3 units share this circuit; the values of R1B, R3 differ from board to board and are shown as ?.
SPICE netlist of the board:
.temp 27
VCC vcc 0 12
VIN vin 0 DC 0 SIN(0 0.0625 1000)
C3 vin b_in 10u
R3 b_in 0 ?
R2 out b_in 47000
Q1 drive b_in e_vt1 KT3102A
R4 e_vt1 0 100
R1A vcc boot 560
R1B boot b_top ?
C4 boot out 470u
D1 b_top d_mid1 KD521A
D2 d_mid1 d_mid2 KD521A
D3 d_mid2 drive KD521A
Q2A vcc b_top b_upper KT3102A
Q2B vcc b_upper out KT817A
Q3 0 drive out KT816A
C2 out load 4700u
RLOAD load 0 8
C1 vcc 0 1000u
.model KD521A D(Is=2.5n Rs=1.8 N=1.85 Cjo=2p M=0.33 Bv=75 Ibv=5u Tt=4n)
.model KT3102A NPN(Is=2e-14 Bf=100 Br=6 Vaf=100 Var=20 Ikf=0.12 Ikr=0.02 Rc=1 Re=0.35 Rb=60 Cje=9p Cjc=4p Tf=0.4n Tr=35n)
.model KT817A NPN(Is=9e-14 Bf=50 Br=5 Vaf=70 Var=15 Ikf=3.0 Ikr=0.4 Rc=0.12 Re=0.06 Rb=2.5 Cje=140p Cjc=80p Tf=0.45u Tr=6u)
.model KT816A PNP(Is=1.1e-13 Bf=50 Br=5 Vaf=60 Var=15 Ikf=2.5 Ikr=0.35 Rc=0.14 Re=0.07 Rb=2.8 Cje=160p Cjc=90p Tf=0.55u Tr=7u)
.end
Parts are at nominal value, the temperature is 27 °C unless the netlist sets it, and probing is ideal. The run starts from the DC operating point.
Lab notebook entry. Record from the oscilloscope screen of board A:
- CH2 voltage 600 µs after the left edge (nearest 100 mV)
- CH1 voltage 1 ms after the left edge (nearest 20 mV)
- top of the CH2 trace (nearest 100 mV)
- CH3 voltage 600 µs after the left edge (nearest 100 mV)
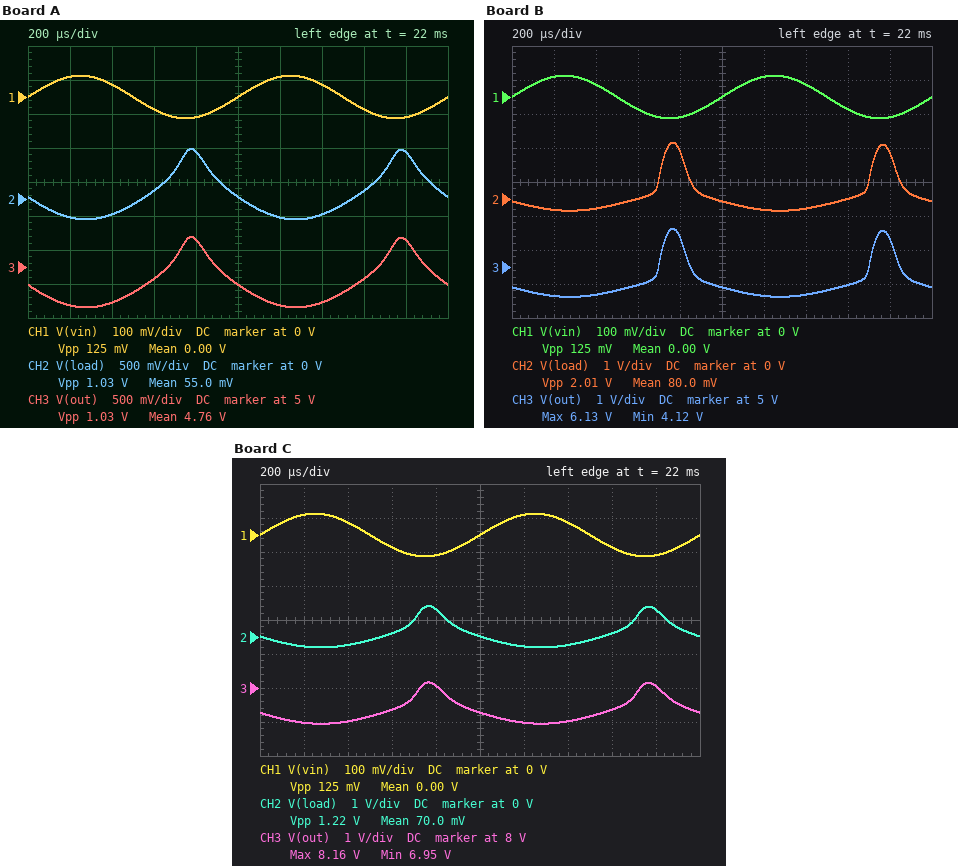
100 mV
0 V
700 mV
4.8 V
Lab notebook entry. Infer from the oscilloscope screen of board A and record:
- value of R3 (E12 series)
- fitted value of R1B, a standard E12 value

18 kΩ
2.2 kΩ
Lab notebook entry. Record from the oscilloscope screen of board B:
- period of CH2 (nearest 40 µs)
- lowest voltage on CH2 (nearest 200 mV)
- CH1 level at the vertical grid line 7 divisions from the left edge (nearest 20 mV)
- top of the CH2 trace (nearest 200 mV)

1.00 ms
-400 mV
40 mV
1.6 V
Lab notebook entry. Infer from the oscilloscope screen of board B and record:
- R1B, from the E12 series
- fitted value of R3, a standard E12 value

3.9 kΩ
15 kΩ
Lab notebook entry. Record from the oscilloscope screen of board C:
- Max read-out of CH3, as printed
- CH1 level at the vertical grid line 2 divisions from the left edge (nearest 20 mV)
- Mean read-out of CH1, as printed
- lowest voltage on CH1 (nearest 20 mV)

8.16 V
40 mV
0.00 V
-60 mV
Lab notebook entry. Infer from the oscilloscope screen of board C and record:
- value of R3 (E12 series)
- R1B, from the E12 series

8.2 kΩ
1.2 kΩ
